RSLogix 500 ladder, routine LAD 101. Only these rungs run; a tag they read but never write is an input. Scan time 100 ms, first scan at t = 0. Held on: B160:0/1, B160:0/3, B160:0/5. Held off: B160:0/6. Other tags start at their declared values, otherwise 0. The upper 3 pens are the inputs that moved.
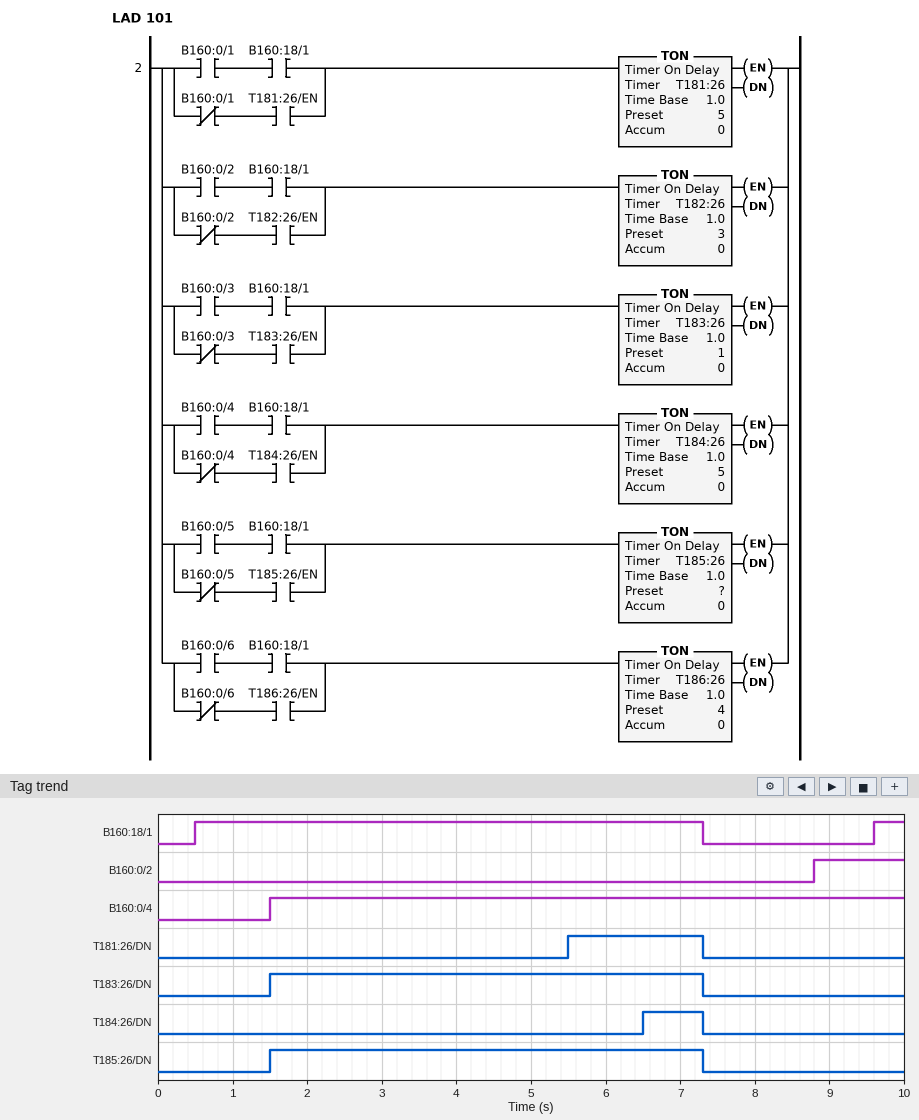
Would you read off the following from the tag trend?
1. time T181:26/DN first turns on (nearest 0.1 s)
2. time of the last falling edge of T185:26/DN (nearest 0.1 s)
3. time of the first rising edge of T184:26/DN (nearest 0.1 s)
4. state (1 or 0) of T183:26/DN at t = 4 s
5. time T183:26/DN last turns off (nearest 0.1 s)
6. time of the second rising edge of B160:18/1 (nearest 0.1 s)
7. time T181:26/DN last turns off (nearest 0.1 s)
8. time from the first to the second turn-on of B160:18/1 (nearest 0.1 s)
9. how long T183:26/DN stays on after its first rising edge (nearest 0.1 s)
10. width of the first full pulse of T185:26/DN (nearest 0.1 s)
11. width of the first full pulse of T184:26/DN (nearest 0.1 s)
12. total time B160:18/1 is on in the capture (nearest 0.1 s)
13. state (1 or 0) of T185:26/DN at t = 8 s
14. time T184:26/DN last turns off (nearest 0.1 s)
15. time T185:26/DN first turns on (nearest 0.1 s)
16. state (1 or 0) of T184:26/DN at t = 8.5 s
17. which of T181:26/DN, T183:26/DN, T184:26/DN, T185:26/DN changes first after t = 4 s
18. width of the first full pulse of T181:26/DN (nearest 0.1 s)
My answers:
5.5 s
7.3 s
6.5 s
1
7.3 s
9.6 s
7.3 s
9.1 s
5.8 s
5.8 s
0.8 s
7.2 s
0
7.3 s
1.5 s
0
T181:26/DN
1.8 s
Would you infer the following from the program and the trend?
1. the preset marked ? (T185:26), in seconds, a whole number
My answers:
1 s
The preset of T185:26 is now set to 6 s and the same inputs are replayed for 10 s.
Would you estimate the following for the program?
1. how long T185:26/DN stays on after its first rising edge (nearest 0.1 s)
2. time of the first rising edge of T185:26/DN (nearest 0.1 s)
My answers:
0.8 s
6.5 s
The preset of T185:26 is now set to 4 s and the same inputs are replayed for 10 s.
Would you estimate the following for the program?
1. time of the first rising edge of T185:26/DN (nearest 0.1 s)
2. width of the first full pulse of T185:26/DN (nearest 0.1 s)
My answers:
4.5 s
2.8 s
